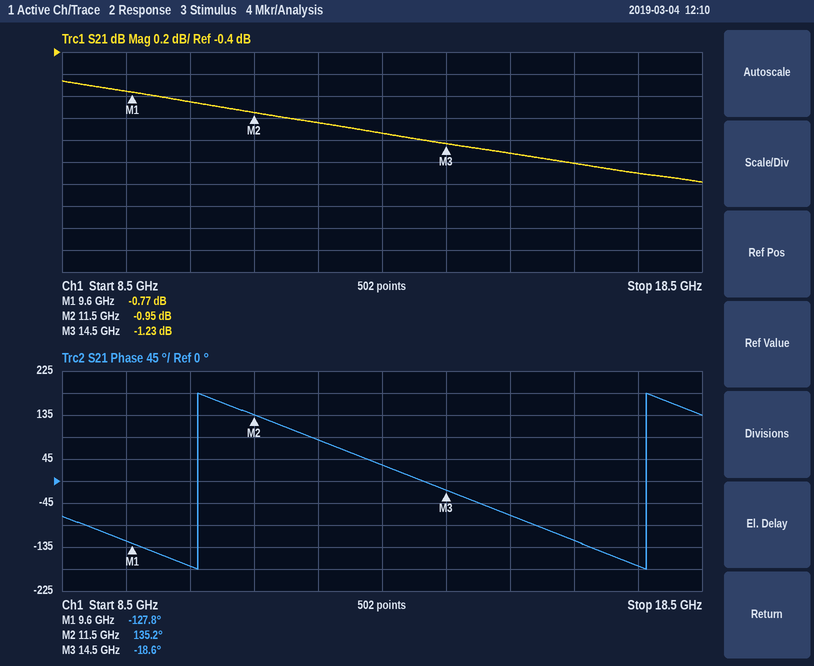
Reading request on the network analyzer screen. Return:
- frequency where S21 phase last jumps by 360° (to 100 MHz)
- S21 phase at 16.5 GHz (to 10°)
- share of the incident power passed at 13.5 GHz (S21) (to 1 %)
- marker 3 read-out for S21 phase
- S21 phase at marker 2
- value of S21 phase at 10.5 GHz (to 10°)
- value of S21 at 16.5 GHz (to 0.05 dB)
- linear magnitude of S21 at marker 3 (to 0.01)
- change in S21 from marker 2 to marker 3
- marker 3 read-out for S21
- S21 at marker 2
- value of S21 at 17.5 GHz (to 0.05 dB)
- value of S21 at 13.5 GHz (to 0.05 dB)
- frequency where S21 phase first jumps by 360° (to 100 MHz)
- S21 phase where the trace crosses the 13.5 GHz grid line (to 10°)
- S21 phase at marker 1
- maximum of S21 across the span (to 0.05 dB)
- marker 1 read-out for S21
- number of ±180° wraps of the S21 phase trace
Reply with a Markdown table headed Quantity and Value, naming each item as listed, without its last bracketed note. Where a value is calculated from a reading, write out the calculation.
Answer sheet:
| Quantity | Value |
|---|---|
| frequency where S21 phase last jumps by 360° | 17.6 GHz |
| S21 phase at 16.5 GHz | -120° |
| share of the incident power passed at 13.5 GHz (S21) | 10^(-1.15/10) ≈ 77 % |
| marker 3 read-out for S21 phase | -18.6° |
| S21 phase at marker 2 | 135.2° |
| value of S21 phase at 10.5 GHz | -170° |
| value of S21 at 16.5 GHz | -1.40 dB |
| linear magnitude of S21 at marker 3 | 10^(-1.23/20) ≈ 0.87 |
| change in S21 from marker 2 to marker 3 | -1.23 − (-0.95) = -0.28 dB |
| marker 3 read-out for S21 | -1.23 dB |
| S21 at marker 2 | -0.95 dB |
| value of S21 at 17.5 GHz | -1.50 dB |
| value of S21 at 13.5 GHz | -1.15 dB |
| frequency where S21 phase first jumps by 360° | 10.6 GHz |
| S21 phase where the trace crosses the 13.5 GHz grid line | 30° |
| S21 phase at marker 1 | -127.8° |
| maximum of S21 across the span | -0.65 dB |
| marker 1 read-out for S21 | -0.77 dB |
| number of ±180° wraps of the S21 phase trace | 2 |
